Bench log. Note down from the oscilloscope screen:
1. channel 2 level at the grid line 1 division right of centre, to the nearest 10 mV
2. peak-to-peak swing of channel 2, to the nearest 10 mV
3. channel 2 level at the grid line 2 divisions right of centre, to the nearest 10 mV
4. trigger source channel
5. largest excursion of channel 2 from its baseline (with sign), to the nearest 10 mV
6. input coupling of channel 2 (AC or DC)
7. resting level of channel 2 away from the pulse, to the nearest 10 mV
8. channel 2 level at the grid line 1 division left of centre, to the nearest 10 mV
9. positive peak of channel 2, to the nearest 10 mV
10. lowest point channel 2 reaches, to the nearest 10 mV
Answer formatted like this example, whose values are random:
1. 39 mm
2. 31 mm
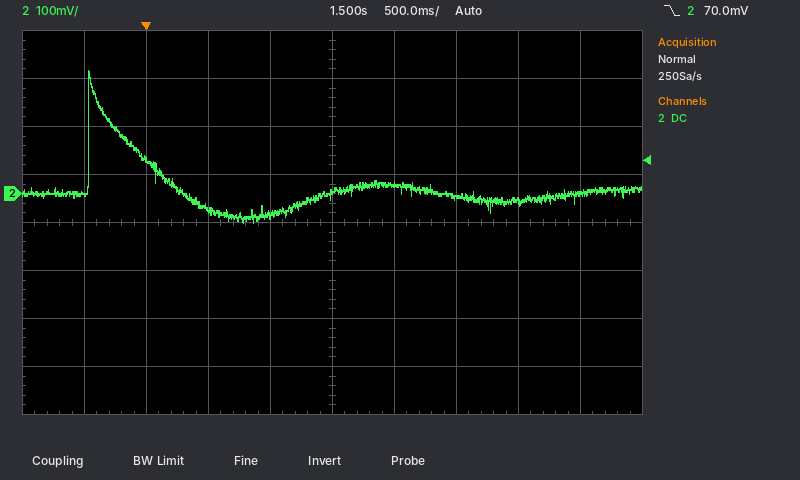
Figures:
1. 20 mV
2. 320 mV
3. -10 mV
4. channel 2
5. +260 mV
6. DC
7. 0 mV
8. -40 mV
9. 260 mV
10. -60 mV
